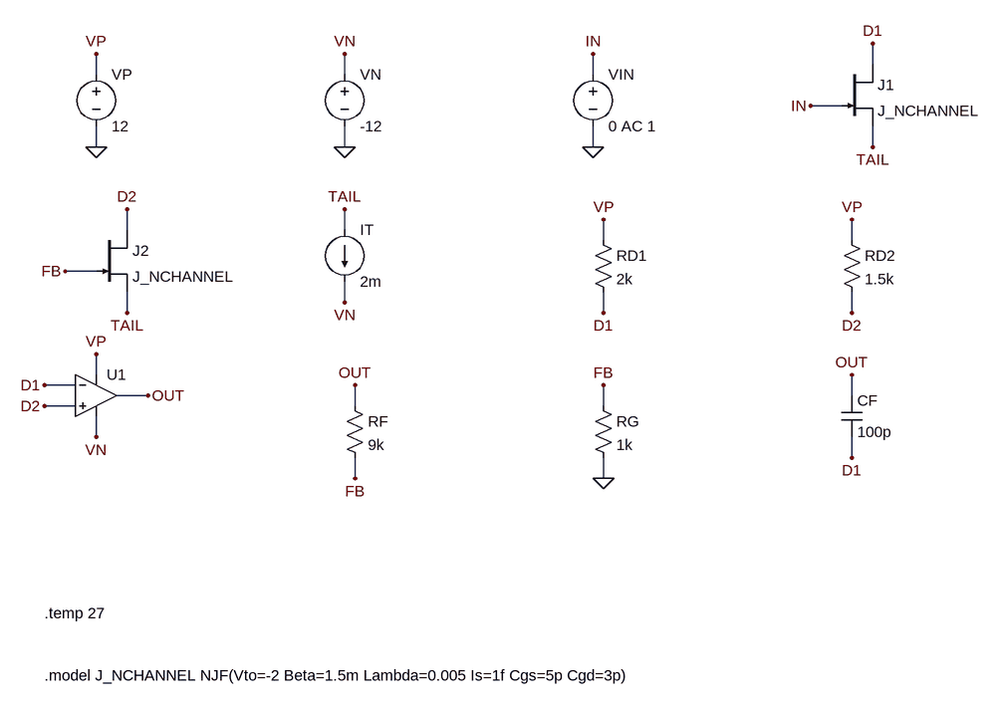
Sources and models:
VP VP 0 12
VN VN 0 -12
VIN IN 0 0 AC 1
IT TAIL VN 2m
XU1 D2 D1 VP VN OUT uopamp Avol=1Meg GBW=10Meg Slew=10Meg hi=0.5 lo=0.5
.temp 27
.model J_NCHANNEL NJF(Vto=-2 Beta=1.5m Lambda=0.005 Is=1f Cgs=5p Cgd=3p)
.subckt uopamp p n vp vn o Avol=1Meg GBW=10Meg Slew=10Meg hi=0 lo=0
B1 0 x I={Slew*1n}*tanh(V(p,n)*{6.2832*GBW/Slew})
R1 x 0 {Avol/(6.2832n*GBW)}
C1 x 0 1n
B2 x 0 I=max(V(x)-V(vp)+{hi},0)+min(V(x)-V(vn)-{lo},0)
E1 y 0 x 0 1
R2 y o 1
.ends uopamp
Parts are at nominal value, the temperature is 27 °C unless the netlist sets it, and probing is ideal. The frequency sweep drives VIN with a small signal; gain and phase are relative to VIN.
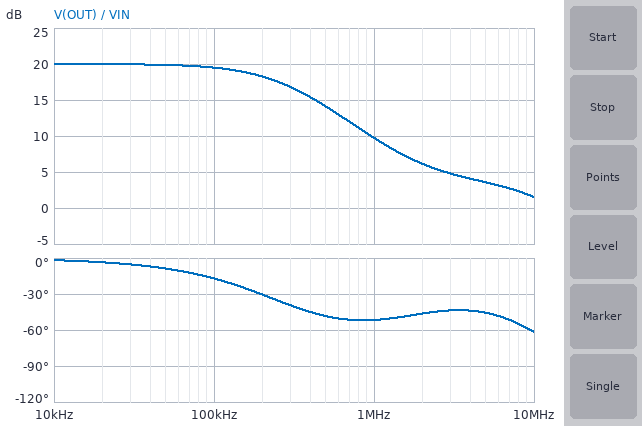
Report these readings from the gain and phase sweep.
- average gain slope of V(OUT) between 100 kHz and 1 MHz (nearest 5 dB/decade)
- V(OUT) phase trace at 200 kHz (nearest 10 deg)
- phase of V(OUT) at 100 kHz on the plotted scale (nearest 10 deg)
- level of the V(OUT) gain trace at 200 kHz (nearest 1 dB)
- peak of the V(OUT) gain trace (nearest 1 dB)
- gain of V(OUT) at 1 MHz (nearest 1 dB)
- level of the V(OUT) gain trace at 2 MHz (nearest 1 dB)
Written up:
-10 dB/decade
-30 deg
-20 deg
18 dB
20 dB
10 dB
6 dB
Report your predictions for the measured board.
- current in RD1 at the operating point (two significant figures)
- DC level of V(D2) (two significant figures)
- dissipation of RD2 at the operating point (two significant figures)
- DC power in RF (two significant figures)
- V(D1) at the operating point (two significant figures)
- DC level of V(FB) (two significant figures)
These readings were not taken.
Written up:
860 µA
10 V
2.0 mW
120 µW
10 V
110 mV
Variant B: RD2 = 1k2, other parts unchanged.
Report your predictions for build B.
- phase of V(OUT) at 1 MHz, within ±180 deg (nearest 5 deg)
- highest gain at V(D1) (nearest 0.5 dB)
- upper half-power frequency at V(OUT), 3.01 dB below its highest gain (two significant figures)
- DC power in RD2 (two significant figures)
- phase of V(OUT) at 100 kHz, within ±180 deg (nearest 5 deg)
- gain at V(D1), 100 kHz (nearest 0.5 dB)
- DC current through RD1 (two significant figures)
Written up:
-55 deg
0.5 dB
260 kHz
1.9 mW
-20 deg
-8.5 dB
750 µA
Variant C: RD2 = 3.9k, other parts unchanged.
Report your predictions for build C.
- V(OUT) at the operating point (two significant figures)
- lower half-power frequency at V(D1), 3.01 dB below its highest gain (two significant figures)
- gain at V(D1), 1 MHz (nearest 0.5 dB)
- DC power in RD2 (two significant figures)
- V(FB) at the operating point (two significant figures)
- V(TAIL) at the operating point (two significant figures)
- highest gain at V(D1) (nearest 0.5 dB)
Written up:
-2.6 V
360 kHz
9.0 dB
1.8 mW
-260 mV
1.1 V
9.5 dB
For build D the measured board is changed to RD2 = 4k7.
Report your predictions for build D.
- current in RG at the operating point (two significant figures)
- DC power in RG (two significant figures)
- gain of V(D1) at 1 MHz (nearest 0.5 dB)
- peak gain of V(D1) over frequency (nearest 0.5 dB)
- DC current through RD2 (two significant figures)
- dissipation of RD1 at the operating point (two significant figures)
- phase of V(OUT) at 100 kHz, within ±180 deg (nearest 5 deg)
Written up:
330 µA
110 µW
10.0 dB
10.5 dB
600 µA
3.9 mW
-10 deg
